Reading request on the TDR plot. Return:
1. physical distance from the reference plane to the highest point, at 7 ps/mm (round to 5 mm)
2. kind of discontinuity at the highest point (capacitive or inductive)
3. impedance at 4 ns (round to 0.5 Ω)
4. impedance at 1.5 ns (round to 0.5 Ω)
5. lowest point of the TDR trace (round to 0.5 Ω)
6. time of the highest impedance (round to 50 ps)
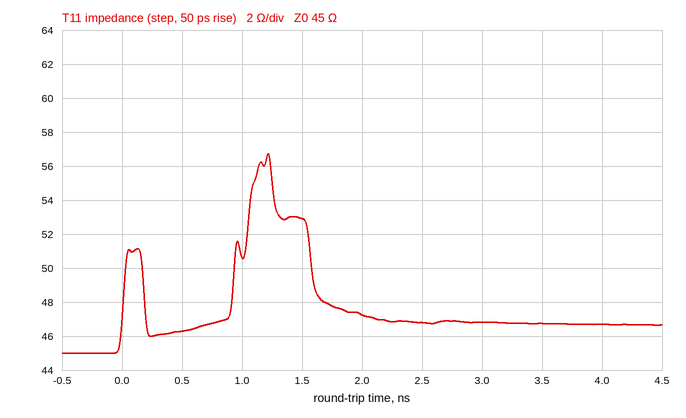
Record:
85 mm
inductive
46.5 Ω
53.0 Ω
45.0 Ω
1.20 ns
